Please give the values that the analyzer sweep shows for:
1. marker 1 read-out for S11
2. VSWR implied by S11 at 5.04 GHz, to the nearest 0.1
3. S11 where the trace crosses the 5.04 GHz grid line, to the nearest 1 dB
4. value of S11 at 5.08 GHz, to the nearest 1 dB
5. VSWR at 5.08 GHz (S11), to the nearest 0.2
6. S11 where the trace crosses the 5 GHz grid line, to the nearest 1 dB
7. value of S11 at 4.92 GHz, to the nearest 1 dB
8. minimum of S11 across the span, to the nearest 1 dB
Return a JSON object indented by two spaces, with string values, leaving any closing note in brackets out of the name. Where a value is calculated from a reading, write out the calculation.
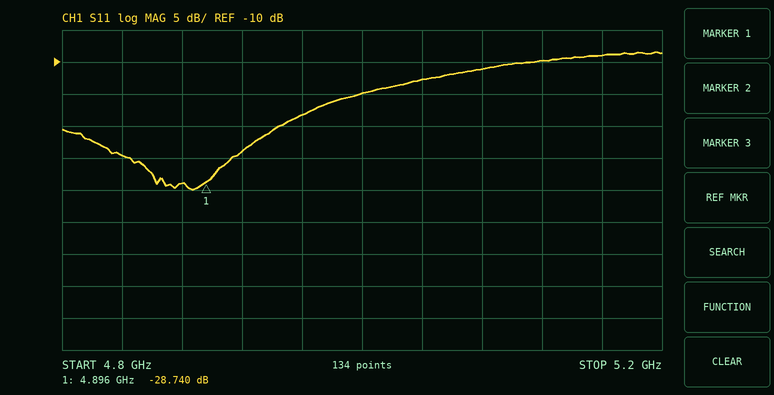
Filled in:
{
  "marker 1 read-out for S11": "-28.740 dB",
  "VSWR implied by S11 at 5.04 GHz, to the nearest 0.1": "|Γ| = 10^(-13/20) = 0.2239; VSWR = (1 + 0.2239)/(1 − 0.2239) ≈ 1.6",
  "S11 where the trace crosses the 5.04 GHz grid line, to the nearest 1 dB": "-13 dB",
  "value of S11 at 5.08 GHz, to the nearest 1 dB": "-11 dB",
  "VSWR at 5.08 GHz (S11), to the nearest 0.2": "|Γ| = 10^(-11/20) = 0.2818; VSWR = (1 + 0.2818)/(1 − 0.2818) ≈ 1.8",
  "S11 where the trace crosses the 5 GHz grid line, to the nearest 1 dB": "-15 dB",
  "value of S11 at 4.92 GHz, to the nearest 1 dB": "-24 dB",
  "minimum of S11 across the span, to the nearest 1 dB": "-30 dB"
}
